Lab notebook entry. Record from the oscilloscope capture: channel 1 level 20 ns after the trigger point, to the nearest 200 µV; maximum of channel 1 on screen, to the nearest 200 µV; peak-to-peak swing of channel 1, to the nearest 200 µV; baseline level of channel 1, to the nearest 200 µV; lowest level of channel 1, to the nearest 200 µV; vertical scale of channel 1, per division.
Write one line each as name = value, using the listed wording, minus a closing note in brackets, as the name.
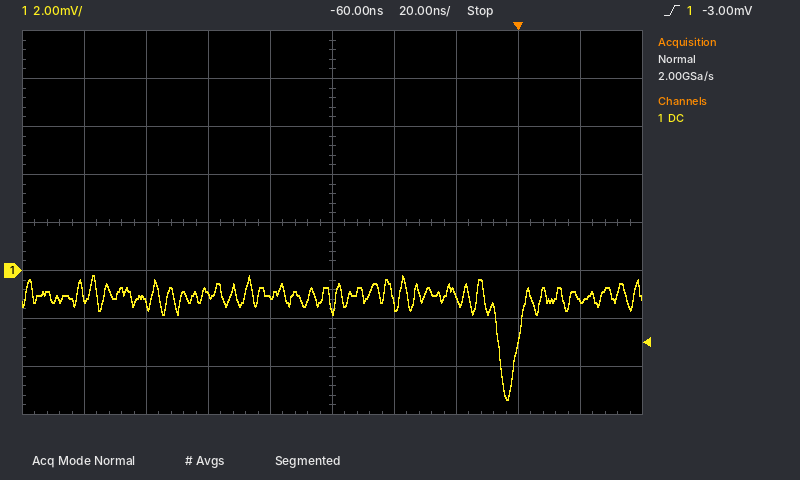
channel 1 level 20 ns after the trigger point, to the nearest 200 µV = -1.2 mV
maximum of channel 1 on screen, to the nearest 200 µV = -200 µV
peak-to-peak swing of channel 1, to the nearest 200 µV = 5.2 mV
baseline level of channel 1, to the nearest 200 µV = -1.0 mV
lowest level of channel 1, to the nearest 200 µV = -5.4 mV
vertical scale of channel 1, per division = 2 mV
